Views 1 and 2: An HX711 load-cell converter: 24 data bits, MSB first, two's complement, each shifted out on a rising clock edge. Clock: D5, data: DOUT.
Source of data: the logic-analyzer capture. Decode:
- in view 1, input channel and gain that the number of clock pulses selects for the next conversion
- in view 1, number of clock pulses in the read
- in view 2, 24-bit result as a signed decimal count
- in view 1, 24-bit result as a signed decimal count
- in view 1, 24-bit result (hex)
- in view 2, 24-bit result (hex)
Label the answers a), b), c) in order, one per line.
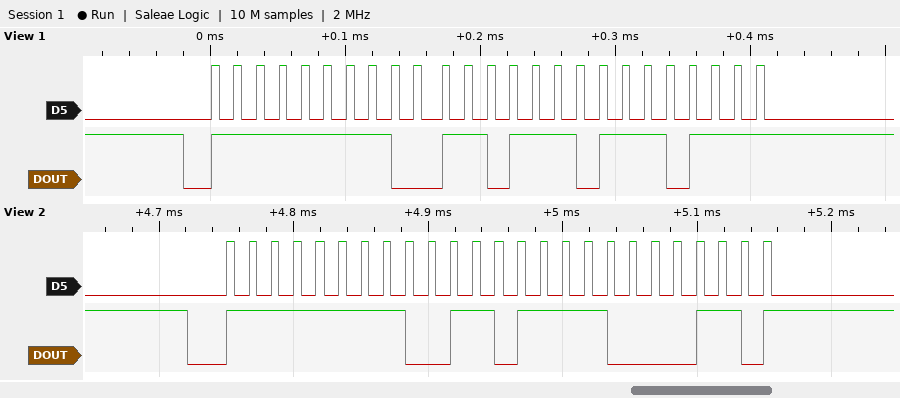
a) channel A, gain 128
b) 25
c) -51322
d) -51337
e) 0xFF3777
f) 0xFF3786
